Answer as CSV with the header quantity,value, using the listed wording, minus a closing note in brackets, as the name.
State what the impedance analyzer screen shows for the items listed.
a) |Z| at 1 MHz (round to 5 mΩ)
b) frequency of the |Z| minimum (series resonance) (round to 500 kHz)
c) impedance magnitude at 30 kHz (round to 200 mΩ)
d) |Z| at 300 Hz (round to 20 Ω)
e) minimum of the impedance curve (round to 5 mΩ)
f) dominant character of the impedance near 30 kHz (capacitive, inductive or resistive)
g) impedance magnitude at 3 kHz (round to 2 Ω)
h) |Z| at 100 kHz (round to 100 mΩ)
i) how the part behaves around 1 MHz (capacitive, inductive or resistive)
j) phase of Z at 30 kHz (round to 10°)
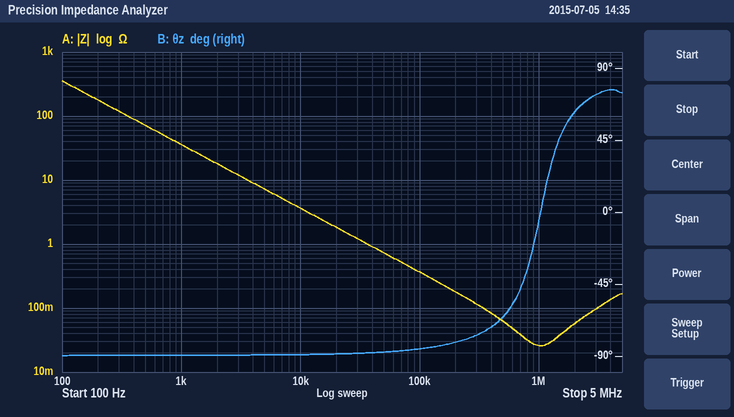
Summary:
quantity,value
|Z| at 1 MHz,25 mΩ
frequency of the |Z| minimum (series resonance),1.0 MHz
impedance magnitude at 30 kHz,1.2 Ω
|Z| at 300 Hz,120 Ω
minimum of the impedance curve,25 mΩ
dominant character of the impedance near 30 kHz,capacitive
impedance magnitude at 3 kHz,12 Ω
|Z| at 100 kHz,400 mΩ
how the part behaves around 1 MHz,resistive
phase of Z at 30 kHz,-90°
